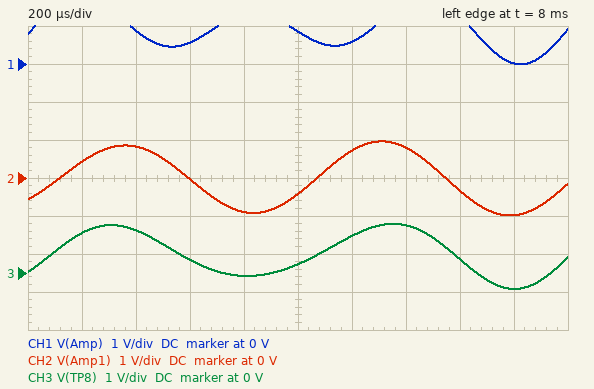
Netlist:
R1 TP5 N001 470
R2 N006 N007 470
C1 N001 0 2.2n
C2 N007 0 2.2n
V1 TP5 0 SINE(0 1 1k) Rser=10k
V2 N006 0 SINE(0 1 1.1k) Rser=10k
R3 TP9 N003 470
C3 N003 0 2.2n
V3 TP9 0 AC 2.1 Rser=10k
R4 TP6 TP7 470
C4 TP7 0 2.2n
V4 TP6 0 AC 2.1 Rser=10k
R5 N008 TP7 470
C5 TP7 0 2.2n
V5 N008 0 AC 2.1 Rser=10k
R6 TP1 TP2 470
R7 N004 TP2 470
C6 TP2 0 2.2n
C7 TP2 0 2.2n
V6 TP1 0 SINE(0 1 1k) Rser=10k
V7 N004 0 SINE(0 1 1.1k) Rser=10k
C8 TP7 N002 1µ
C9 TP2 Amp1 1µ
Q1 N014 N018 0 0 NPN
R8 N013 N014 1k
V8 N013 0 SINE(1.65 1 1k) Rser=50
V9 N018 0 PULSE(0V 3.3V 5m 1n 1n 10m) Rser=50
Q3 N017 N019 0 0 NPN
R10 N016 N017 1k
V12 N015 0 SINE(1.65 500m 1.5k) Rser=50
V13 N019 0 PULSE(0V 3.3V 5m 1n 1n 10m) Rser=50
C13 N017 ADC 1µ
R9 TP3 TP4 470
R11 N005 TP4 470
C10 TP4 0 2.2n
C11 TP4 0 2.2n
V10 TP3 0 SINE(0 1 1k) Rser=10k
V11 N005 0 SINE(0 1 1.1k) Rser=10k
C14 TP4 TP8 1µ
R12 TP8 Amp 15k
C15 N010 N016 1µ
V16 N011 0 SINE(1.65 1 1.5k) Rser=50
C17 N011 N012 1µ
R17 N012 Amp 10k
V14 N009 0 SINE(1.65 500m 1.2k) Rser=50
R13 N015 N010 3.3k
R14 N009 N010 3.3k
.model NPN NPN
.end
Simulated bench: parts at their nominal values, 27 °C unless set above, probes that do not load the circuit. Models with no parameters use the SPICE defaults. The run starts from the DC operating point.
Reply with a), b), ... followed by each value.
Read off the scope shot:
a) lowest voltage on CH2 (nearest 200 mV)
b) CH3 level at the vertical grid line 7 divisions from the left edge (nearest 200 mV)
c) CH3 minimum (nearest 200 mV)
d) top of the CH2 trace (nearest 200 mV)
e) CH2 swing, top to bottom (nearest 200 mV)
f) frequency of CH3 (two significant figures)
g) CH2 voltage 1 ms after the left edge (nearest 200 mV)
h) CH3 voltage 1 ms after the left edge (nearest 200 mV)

a) -1.0 V
b) 1.2 V
c) -400 mV
d) 1.0 V
e) 2.0 V
f) 1.0 kHz
g) -400 mV
h) 200 mV
